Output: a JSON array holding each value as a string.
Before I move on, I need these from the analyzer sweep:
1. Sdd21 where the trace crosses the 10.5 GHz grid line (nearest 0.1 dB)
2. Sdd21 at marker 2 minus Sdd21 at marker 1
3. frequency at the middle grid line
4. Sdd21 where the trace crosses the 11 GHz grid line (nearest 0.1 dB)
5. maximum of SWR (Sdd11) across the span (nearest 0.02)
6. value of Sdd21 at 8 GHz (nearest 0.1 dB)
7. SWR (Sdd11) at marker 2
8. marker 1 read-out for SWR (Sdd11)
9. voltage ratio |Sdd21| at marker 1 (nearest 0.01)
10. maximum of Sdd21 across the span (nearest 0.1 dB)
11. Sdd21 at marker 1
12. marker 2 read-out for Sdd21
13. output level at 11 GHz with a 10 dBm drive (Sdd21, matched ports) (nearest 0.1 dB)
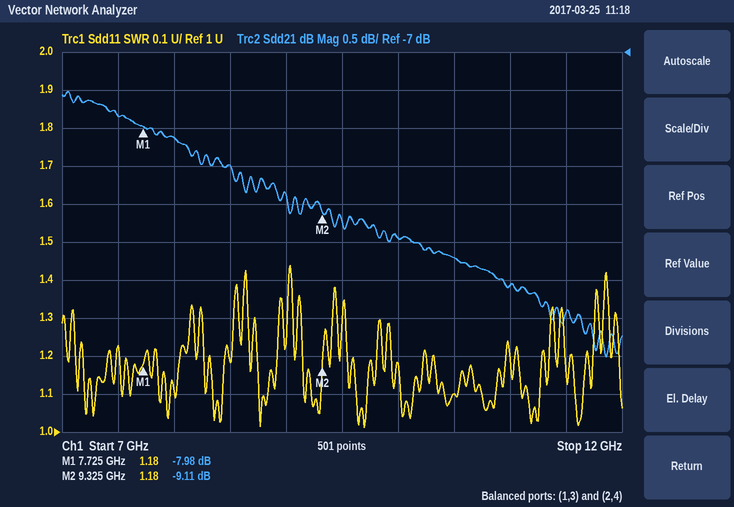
["-9.7 dB", "-1.13 dB", "9.5 GHz", "-10.1 dB", "1.44", "-8.1 dB", "1.18", "1.18", "0.40", "-7.5 dB", "-7.98 dB", "-9.11 dB", "-0.1 dBm"]
